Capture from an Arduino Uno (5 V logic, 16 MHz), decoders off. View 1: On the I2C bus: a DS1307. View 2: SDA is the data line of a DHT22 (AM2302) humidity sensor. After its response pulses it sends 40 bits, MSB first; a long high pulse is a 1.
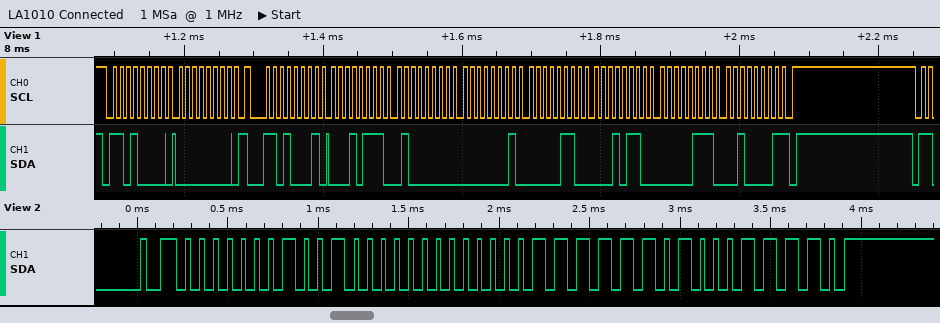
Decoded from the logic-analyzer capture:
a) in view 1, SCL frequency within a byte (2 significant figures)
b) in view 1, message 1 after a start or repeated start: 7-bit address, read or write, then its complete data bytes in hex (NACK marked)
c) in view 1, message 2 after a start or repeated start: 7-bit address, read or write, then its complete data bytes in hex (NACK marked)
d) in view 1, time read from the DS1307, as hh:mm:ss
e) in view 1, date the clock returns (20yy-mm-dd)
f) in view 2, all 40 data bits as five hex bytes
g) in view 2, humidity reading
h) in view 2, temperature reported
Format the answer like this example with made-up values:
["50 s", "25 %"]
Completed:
["100 kHz", "0x68 write: 00", "0x68 read: 17 40 01 06 16 07 21 NACK", "01:40:17", "2021-07-16", "01 20 00 FD 1E", "28.8 %", "25.3 °C"]
